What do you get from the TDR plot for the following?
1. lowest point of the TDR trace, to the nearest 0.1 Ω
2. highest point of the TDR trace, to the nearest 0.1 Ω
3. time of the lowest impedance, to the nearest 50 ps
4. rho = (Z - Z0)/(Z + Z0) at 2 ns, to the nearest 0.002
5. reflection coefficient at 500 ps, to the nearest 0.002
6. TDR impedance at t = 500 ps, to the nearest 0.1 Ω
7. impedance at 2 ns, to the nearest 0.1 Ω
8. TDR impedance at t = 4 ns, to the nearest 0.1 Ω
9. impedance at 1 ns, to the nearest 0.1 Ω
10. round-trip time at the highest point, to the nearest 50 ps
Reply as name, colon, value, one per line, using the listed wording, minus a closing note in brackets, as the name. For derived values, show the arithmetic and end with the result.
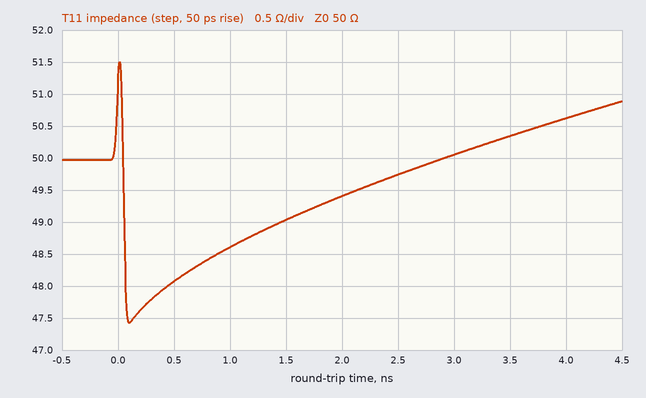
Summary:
lowest point of the TDR trace, to the nearest 0.1 Ω: 47.4 Ω
highest point of the TDR trace, to the nearest 0.1 Ω: 51.5 Ω
time of the lowest impedance, to the nearest 50 ps: 100 ps
rho = (Z - Z0)/(Z + Z0) at 2 ns, to the nearest 0.002: (49.4 − 50)/(49.4 + 50) ≈ -0.006
reflection coefficient at 500 ps, to the nearest 0.002: (48.1 − 50)/(48.1 + 50) ≈ -0.0194, so -0.020 to the nearest 0.002
TDR impedance at t = 500 ps, to the nearest 0.1 Ω: 48.1 Ω
impedance at 2 ns, to the nearest 0.1 Ω: 49.4 Ω
TDR impedance at t = 4 ns, to the nearest 0.1 Ω: 50.6 Ω
impedance at 1 ns, to the nearest 0.1 Ω: 48.6 Ω
round-trip time at the highest point, to the nearest 50 ps: 0 ps
